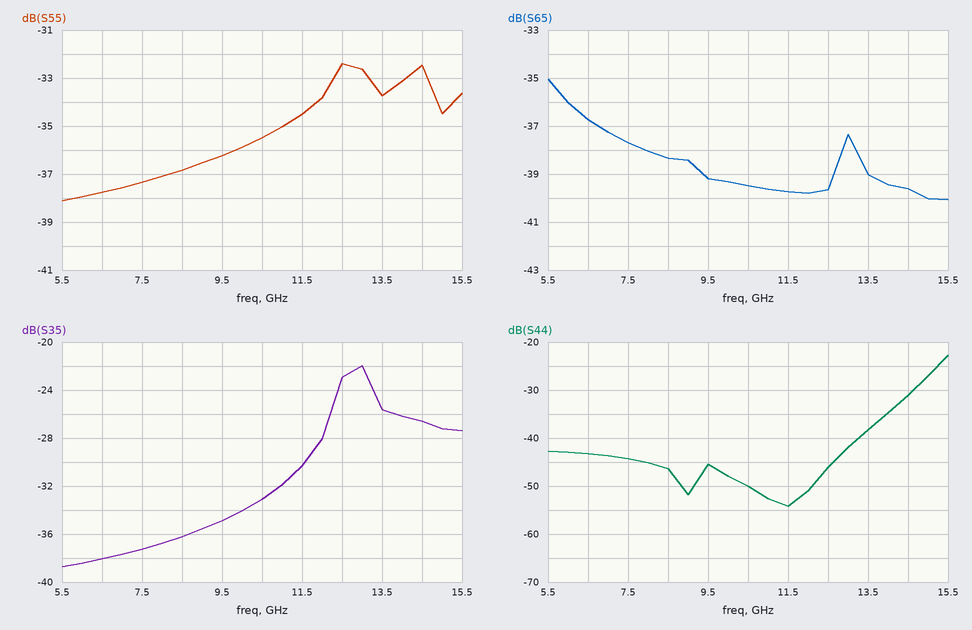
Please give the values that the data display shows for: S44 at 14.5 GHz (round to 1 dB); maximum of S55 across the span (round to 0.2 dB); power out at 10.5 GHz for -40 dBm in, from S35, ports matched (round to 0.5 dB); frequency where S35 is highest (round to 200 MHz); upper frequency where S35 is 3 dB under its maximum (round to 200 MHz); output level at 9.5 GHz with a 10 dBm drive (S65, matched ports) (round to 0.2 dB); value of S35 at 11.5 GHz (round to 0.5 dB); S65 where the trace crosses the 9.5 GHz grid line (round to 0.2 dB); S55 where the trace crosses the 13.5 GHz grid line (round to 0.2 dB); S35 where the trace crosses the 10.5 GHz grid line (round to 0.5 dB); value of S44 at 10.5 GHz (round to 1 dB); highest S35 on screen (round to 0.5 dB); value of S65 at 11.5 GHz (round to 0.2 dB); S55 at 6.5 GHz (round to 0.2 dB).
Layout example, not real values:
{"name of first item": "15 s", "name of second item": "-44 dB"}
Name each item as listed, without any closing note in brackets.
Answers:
{"S44 at 14.5 GHz": "-31 dB", "maximum of S55 across the span": "-32.4 dB", "power out at 10.5 GHz for -40 dBm in, from S35, ports matched": "-73.0 dBm", "frequency where S35 is highest": "13.0 GHz", "upper frequency where S35 is 3 dB under its maximum": "13.4 GHz", "output level at 9.5 GHz with a 10 dBm drive (S65, matched ports)": "-29.2 dBm", "value of S35 at 11.5 GHz": "-30.5 dB", "S65 where the trace crosses the 9.5 GHz grid line": "-39.2 dB", "S55 where the trace crosses the 13.5 GHz grid line": "-33.8 dB", "S35 where the trace crosses the 10.5 GHz grid line": "-33.0 dB", "value of S44 at 10.5 GHz": "-50 dB", "highest S35 on screen": "-22.0 dB", "value of S65 at 11.5 GHz": "-39.8 dB", "S55 at 6.5 GHz": "-37.8 dB"}
